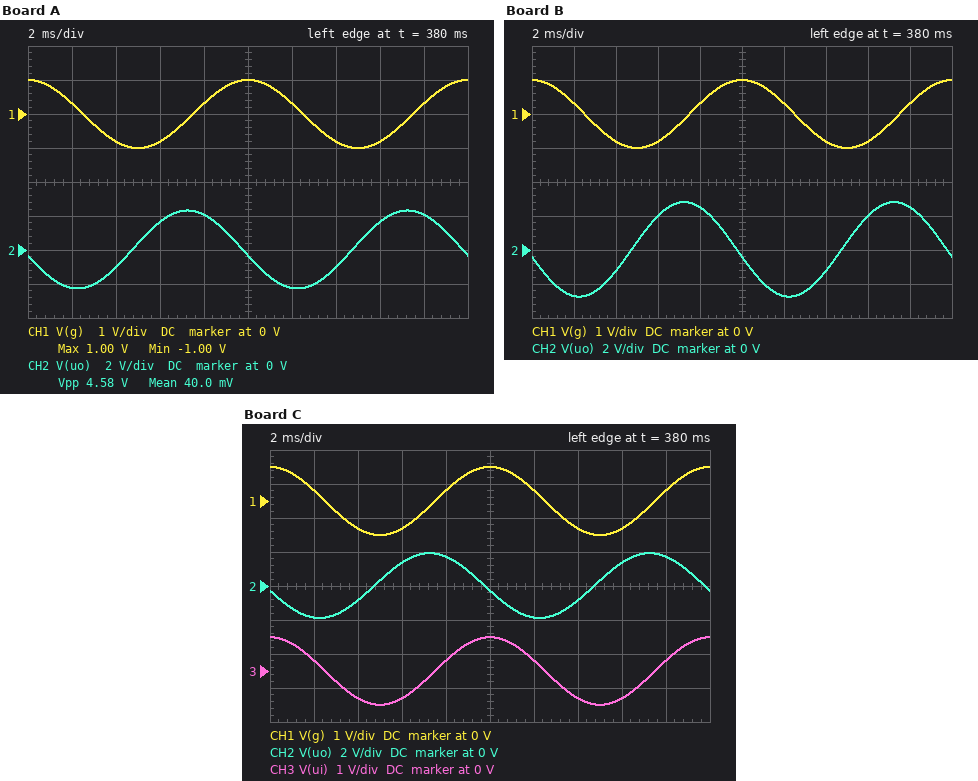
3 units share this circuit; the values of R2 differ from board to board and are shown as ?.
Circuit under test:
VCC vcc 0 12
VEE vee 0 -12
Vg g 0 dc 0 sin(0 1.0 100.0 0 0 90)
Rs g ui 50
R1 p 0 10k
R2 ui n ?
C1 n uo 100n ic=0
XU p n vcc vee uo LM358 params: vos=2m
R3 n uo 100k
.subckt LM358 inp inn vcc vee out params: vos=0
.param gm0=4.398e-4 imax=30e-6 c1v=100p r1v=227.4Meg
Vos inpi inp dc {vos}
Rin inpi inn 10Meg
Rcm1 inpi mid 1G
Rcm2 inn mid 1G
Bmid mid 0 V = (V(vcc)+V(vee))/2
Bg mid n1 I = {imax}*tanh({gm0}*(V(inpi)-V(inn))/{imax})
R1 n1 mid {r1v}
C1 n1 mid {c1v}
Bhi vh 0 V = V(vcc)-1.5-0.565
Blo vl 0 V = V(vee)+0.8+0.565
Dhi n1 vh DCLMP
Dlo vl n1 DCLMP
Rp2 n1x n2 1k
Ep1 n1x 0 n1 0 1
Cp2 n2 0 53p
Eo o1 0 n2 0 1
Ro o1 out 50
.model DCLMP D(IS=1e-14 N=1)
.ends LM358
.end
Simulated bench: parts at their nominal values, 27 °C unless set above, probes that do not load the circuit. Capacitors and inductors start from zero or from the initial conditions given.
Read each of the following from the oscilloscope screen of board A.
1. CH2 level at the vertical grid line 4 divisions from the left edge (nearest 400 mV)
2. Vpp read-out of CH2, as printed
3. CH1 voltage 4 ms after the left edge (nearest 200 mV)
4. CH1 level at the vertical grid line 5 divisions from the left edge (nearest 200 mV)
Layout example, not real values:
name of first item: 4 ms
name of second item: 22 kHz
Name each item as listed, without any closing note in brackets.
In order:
CH2 level at the vertical grid line 4 divisions from the left edge: 2.0 V
Vpp read-out of CH2, as printed: 4.58 V
CH1 voltage 4 ms after the left edge: -800 mV
CH1 level at the vertical grid line 5 divisions from the left edge: 1.0 V
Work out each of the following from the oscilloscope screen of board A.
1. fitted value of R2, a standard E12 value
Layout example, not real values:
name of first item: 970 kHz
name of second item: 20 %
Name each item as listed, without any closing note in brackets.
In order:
fitted value of R2, a standard E12 value: 6.8 kΩ
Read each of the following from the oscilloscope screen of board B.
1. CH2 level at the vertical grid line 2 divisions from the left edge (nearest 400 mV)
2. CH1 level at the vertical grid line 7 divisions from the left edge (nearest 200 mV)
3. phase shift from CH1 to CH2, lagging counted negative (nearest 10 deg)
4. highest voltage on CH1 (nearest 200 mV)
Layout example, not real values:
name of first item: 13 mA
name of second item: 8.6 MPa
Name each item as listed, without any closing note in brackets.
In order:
CH2 level at the vertical grid line 2 divisions from the left edge: -1.2 V
CH1 level at the vertical grid line 7 divisions from the left edge: -800 mV
phase shift from CH1 to CH2, lagging counted negative: 100 deg
highest voltage on CH1: 1.0 V
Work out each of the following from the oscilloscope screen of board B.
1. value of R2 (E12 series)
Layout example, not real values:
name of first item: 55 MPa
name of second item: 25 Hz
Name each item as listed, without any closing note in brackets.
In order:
value of R2: 5.6 kΩ
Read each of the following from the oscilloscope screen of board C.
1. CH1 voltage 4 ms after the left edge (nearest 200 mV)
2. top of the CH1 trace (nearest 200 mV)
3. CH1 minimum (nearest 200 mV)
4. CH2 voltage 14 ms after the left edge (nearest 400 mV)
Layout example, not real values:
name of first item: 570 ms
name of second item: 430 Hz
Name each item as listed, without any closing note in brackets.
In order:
CH1 voltage 4 ms after the left edge: -800 mV
top of the CH1 trace: 1.0 V
CH1 minimum: -1.0 V
CH2 voltage 14 ms after the left edge: -800 mV
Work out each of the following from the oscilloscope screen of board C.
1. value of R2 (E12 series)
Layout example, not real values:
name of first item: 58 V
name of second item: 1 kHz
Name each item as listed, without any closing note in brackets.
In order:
value of R2: 8.2 kΩ
